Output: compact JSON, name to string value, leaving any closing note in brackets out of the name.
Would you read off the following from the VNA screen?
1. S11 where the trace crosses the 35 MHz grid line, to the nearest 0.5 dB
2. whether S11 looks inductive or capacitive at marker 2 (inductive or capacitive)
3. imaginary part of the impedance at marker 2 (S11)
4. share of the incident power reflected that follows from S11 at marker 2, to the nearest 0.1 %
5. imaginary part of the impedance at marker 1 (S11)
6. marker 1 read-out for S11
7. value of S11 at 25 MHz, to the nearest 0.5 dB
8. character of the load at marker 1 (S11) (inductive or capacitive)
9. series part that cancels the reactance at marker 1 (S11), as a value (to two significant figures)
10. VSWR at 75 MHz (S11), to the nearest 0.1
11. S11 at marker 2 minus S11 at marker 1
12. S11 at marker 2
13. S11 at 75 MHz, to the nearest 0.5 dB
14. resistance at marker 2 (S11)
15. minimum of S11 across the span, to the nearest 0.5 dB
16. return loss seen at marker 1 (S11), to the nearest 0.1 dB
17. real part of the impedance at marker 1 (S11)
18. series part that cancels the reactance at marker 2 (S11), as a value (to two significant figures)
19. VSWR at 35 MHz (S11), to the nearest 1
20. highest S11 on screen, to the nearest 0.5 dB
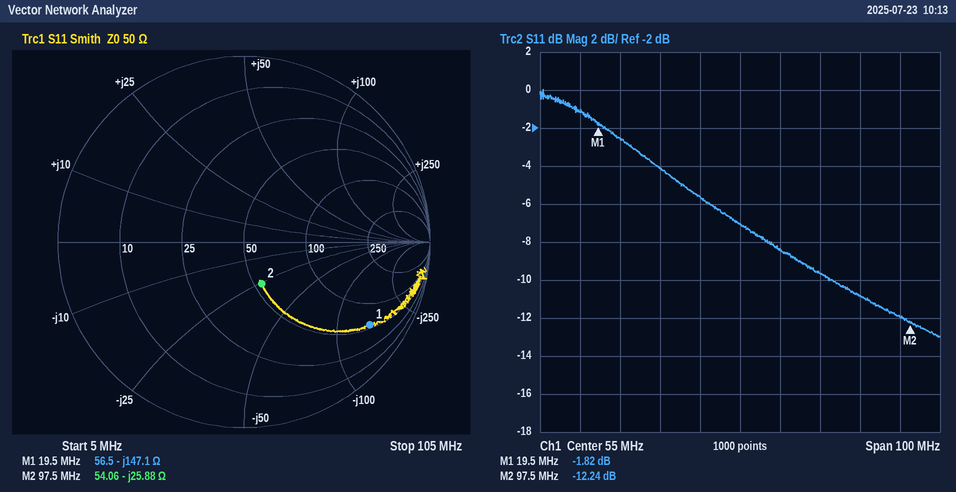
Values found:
{"S11 where the trace crosses the 35 MHz grid line, to the nearest 0.5 dB": "-4.0 dB", "whether S11 looks inductive or capacitive at marker 2": "capacitive", "imaginary part of the impedance at marker 2": "-25.88 Ω", "share of the incident power reflected that follows from S11 at marker 2, to the nearest 0.1 %": "6.0 %", "imaginary part of the impedance at marker 1": "-147.1 Ω", "marker 1 read-out for S11": "-1.82 dB", "value of S11 at 25 MHz, to the nearest 0.5 dB": "-2.5 dB", "character of the load at marker 1 (S11)": "capacitive", "series part that cancels the reactance at marker 1 (S11), as a value": "1.2 µH", "VSWR at 75 MHz (S11), to the nearest 0.1": "2.0", "S11 at marker 2 minus S11 at marker 1": "-10.42 dB", "S11 at marker 2": "-12.24 dB", "S11 at 75 MHz, to the nearest 0.5 dB": "-9.5 dB", "resistance at marker 2": "54.06 Ω", "minimum of S11 across the span, to the nearest 0.5 dB": "-13.0 dB", "return loss seen at marker 1 (S11), to the nearest 0.1 dB": "1.8 dB", "real part of the impedance at marker 1": "56.5 Ω", "series part that cancels the reactance at marker 2 (S11), as a value": "42 nH", "VSWR at 35 MHz (S11), to the nearest 1": "4", "highest S11 on screen, to the nearest 0.5 dB": "0.0 dB"}
